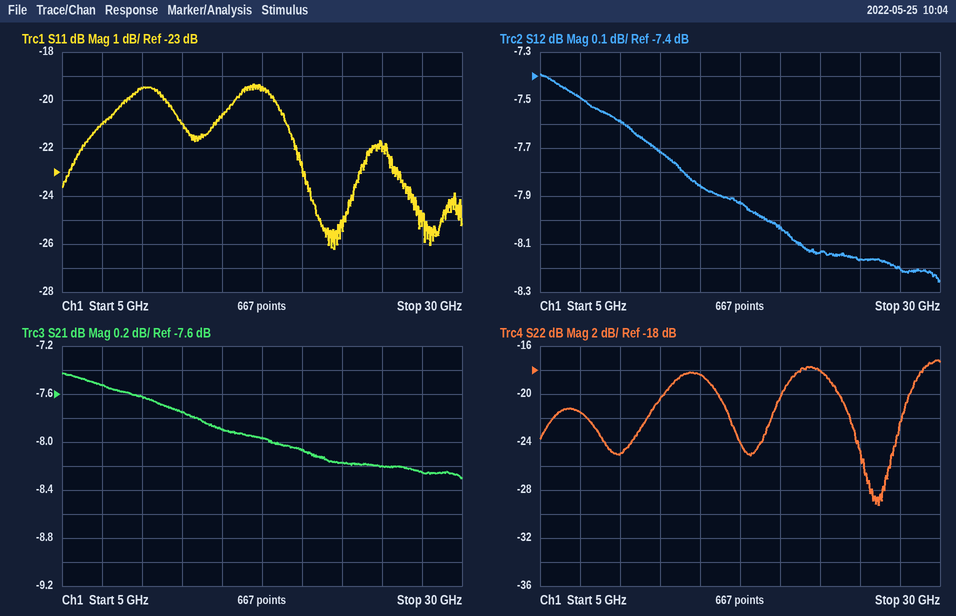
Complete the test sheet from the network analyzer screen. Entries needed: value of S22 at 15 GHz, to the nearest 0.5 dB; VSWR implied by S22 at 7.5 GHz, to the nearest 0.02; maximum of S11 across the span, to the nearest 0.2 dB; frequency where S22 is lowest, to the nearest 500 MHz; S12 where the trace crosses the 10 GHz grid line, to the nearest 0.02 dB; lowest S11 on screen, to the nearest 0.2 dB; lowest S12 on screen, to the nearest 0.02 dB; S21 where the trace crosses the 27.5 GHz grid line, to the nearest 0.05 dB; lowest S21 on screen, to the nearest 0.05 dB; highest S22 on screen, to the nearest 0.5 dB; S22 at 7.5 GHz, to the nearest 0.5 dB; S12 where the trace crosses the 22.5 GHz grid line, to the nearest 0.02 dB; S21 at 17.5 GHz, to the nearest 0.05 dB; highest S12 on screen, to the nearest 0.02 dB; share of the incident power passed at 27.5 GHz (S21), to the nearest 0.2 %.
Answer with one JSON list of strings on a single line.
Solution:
["-18.5 dB", "1.18", "-19.4 dB", "26.0 GHz", "-7.58 dB", "-26.2 dB", "-8.26 dB", "-8.25 dB", "-8.30 dB", "-17.0 dB", "-21.5 dB", "-8.14 dB", "-7.95 dB", "-7.40 dB", "15.0 %"]
